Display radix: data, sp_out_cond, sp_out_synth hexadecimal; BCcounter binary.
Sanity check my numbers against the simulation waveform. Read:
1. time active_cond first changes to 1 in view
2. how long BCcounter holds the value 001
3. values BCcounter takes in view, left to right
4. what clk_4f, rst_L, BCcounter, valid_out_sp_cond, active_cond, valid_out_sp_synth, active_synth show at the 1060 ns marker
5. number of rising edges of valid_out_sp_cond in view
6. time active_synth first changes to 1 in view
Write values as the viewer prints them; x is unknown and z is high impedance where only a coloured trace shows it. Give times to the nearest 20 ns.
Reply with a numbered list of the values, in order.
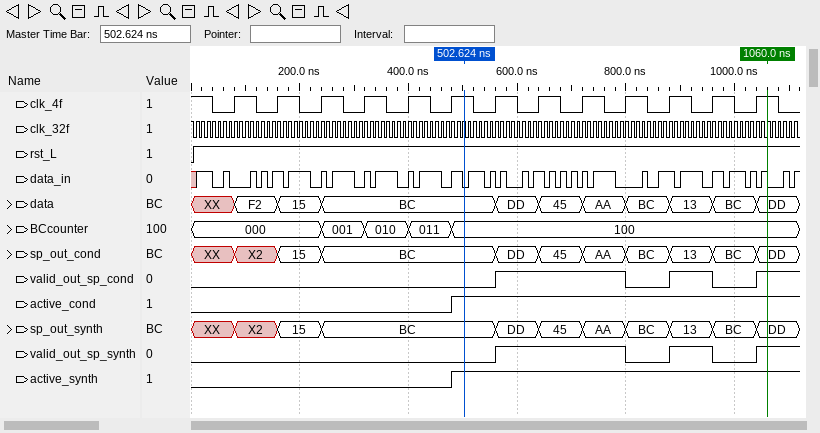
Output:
1. 480 ns
2. 80 ns
3. 000, 001, 010, 011, 100
4. clk_4f=1, rst_L=1, BCcounter=100, valid_out_sp_cond=1, active_cond=1, valid_out_sp_synth=1, active_synth=1
5. 3
6. 480 ns
